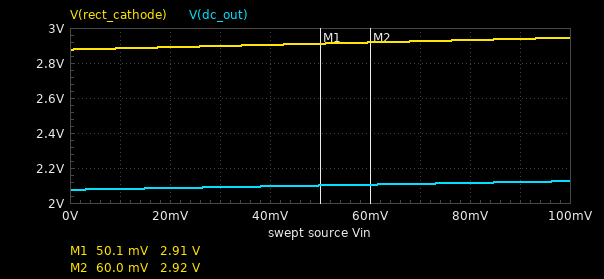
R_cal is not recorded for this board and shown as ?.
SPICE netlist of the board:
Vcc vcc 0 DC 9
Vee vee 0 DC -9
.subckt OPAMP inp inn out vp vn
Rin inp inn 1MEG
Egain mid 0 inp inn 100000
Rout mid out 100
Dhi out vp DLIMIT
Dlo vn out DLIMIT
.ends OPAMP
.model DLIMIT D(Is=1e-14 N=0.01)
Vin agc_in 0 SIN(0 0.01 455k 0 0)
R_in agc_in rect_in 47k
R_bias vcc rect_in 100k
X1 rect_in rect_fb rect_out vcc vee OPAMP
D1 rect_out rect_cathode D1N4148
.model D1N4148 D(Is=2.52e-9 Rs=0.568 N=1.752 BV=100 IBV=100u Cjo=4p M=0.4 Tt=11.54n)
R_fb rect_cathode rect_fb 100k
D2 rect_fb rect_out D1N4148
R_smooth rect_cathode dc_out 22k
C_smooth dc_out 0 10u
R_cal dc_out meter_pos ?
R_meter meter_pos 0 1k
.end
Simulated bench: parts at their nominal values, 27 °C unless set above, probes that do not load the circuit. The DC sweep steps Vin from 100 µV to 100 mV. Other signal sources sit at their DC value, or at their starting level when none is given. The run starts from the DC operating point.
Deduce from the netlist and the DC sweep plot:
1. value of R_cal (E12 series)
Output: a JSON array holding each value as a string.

["56 kΩ"]
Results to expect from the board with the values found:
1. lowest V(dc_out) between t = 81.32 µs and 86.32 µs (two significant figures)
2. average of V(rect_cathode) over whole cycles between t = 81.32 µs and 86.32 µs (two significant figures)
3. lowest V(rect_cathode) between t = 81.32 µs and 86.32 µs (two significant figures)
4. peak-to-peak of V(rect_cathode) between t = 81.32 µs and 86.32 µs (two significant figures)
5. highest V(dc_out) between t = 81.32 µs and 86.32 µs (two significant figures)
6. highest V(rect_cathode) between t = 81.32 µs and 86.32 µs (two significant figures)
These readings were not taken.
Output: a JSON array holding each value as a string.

["2.1 V", "2.9 V", "2.9 V", "13 mV", "2.1 V", "2.9 V"]
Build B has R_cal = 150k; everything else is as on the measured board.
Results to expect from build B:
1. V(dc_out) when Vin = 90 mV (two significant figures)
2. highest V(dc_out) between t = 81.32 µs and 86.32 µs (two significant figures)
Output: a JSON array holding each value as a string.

["2.6 V", "2.5 V"]
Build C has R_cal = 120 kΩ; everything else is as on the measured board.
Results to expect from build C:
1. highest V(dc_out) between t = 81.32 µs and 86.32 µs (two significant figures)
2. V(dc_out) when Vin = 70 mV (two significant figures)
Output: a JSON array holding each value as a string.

["2.4 V", "2.5 V"]
